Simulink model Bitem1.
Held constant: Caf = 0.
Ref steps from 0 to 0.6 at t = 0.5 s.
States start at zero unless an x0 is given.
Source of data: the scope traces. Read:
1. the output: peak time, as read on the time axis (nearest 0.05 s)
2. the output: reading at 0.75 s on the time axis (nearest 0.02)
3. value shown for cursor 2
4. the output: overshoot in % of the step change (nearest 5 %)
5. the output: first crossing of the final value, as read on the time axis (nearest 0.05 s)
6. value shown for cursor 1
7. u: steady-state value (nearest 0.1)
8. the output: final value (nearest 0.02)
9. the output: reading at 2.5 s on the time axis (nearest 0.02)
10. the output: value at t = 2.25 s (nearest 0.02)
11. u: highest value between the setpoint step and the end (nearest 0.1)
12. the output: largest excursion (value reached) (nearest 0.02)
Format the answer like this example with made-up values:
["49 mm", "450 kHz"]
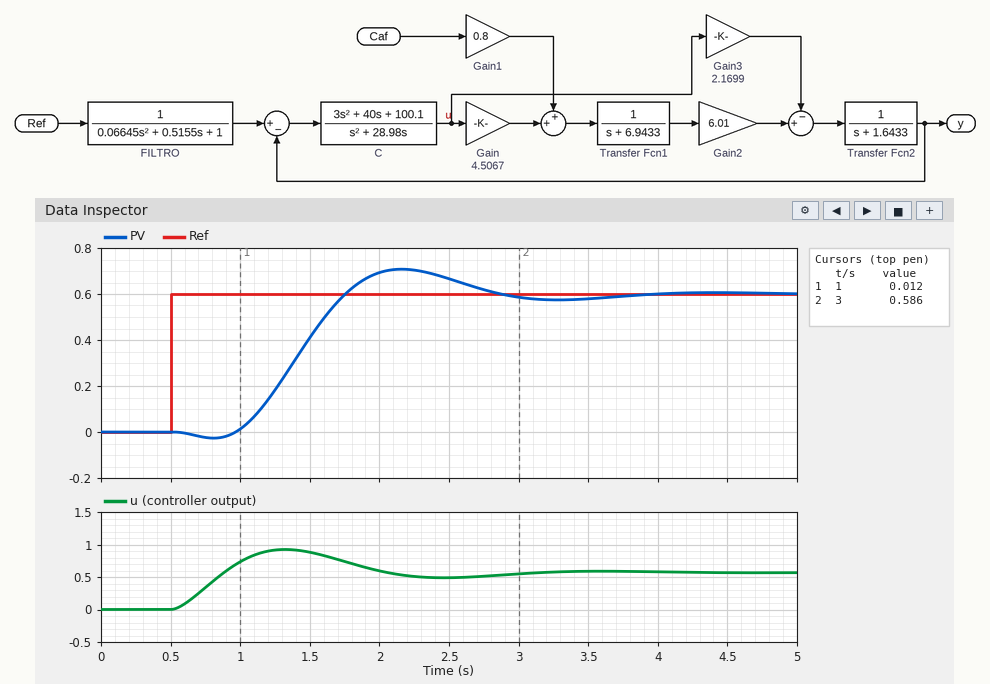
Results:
["2.15 s", "-0.02", "0.586", "20 %", "1.75 s", "0.012", "0.6", "0.60", "0.66", "0.70", "0.9", "0.70"]
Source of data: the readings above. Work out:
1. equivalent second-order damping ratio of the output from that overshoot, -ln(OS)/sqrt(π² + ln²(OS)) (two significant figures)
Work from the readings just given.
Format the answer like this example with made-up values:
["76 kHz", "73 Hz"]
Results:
["0.46"]
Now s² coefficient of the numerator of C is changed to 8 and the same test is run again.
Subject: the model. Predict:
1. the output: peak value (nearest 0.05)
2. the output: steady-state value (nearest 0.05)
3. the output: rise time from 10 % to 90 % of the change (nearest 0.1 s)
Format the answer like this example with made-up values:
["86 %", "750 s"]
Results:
["0.65", "0.60", "0.8 s"]
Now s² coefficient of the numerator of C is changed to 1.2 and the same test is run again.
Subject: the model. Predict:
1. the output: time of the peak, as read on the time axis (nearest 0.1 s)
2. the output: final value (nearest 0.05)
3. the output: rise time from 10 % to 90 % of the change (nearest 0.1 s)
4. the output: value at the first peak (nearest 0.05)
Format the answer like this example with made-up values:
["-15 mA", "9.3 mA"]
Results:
["2.1 s", "0.60", "0.5 s", "0.75"]
